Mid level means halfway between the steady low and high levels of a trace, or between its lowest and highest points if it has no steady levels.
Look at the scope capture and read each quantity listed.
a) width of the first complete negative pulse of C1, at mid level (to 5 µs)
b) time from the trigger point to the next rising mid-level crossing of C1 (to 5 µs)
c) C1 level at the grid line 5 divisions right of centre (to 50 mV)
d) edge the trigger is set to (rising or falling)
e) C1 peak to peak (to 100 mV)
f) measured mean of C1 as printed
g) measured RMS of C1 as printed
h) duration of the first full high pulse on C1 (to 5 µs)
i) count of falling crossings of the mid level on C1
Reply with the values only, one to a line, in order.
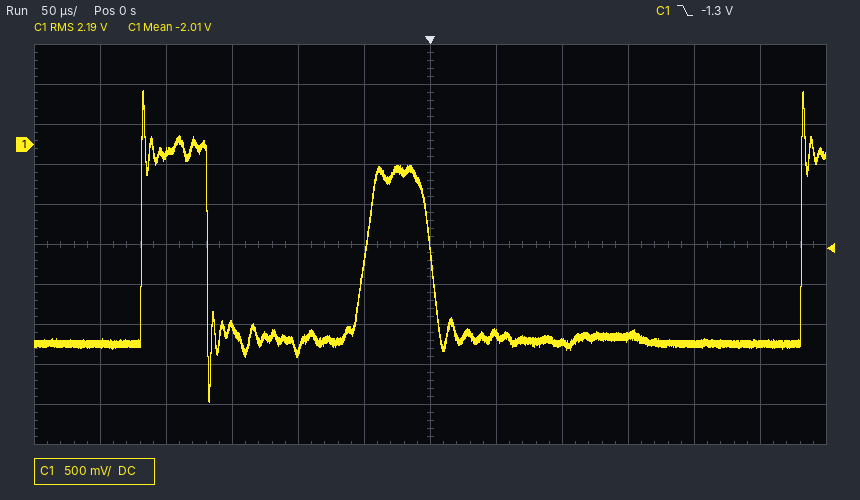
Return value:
120 µs
280 µs
-2.50 V
falling
3.90 V
-2.01 V
2.19 V
50 µs
2
